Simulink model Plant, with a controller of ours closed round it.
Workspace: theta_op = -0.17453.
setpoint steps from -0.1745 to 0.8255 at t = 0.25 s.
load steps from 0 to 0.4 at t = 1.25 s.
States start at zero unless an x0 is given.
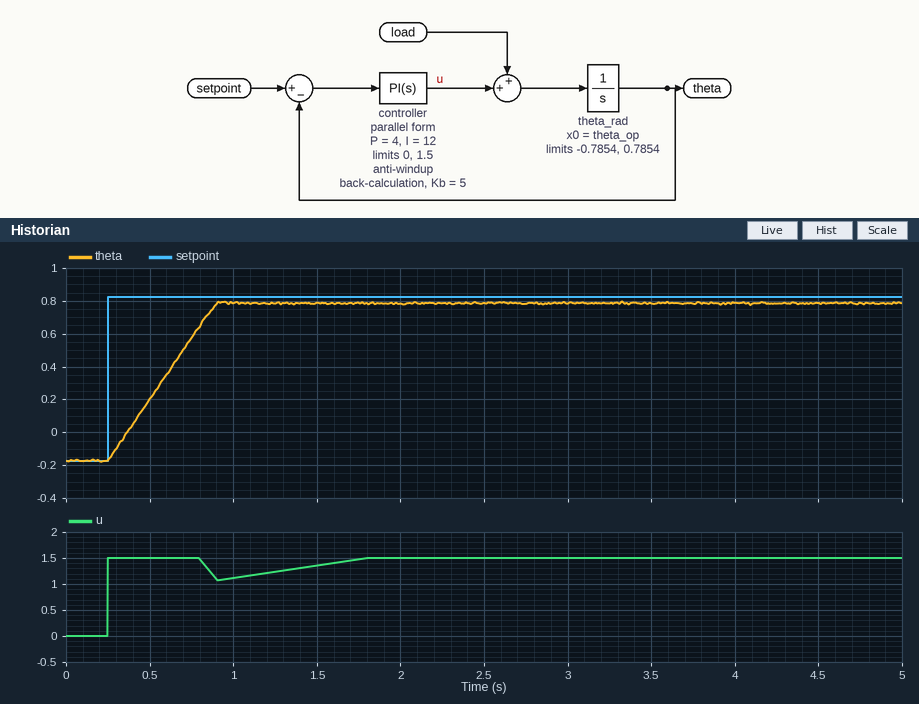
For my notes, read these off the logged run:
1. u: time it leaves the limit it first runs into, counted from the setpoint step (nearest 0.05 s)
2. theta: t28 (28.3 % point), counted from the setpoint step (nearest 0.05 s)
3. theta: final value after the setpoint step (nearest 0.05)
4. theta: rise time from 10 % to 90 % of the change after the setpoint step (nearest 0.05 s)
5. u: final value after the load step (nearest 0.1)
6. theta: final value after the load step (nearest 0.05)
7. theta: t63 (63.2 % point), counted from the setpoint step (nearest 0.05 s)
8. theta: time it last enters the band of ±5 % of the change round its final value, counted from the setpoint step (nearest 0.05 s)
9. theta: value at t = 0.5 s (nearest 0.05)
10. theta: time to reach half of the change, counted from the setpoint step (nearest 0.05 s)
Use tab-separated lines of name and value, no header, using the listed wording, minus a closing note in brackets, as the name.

u: time it leaves the limit it first runs into, counted from the setpoint step	0.55 s
theta: t28 (28.3 % point), counted from the setpoint step	0.20 s
theta: final value after the setpoint step	0.80
theta: rise time from 10 % to 90 % of the change after the setpoint step	0.50 s
u: final value after the load step	1.5
theta: final value after the load step	0.80
theta: t63 (63.2 % point), counted from the setpoint step	0.40 s
theta: time it last enters the band of ±5 % of the change round its final value, counted from the setpoint step	0.60 s
theta: value at t = 0.5 s	0.20
theta: time to reach half of the change, counted from the setpoint step	0.30 s
